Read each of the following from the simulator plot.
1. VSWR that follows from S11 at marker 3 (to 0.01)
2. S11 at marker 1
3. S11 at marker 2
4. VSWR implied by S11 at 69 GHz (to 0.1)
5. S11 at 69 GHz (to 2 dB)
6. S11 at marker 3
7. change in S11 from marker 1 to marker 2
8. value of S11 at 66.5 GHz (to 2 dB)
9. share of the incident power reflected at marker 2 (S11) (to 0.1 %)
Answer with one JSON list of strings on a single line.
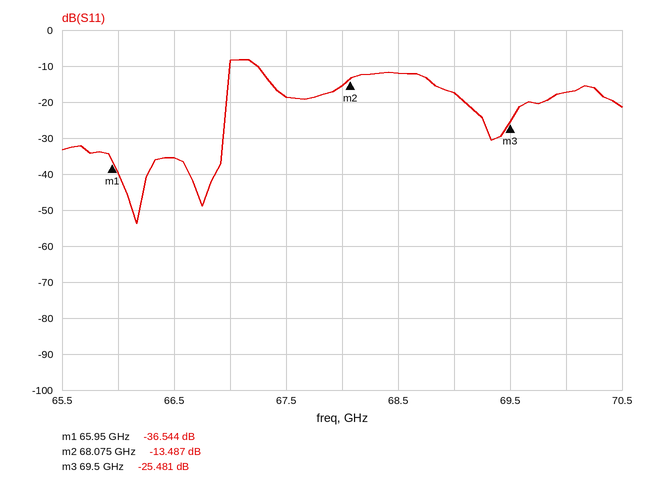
["1.11", "-36.544 dB", "-13.487 dB", "1.3", "-18 dB", "-25.481 dB", "23.057 dB", "-36 dB", "4.5 %"]
